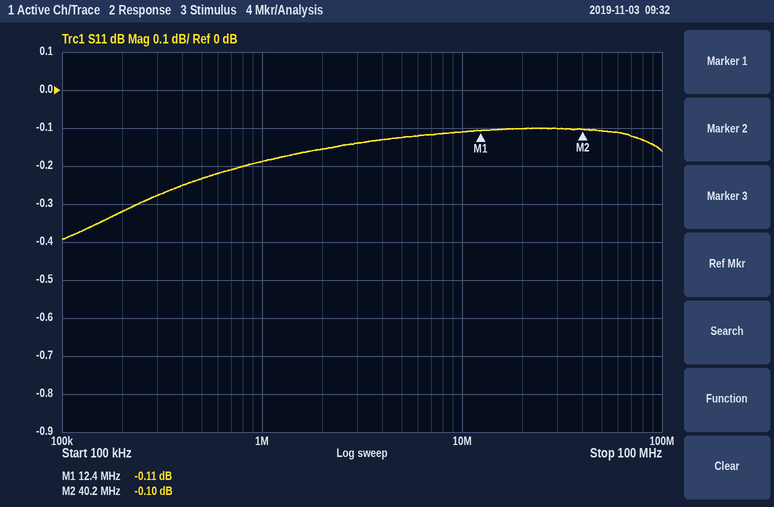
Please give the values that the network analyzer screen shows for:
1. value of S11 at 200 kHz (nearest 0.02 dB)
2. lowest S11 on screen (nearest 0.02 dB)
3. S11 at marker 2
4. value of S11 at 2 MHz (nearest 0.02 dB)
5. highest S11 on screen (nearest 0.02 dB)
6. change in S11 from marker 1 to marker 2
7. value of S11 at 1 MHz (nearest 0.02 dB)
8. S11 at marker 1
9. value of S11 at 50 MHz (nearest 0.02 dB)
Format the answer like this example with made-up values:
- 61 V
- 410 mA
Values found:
- -0.32 dB
- -0.40 dB
- -0.10 dB
- -0.16 dB
- -0.10 dB
- 0.01 dB
- -0.18 dB
- -0.11 dB
- -0.10 dB
